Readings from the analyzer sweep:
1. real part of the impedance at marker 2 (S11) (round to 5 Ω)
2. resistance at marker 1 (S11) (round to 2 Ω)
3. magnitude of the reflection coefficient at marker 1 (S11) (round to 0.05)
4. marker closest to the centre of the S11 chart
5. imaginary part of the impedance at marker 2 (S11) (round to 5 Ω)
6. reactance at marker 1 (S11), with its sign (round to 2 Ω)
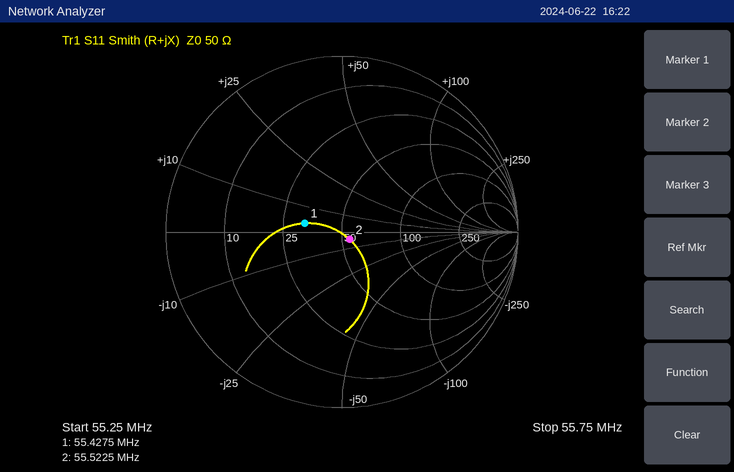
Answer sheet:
55 Ω
32 Ω
0.20
marker 2
-5 Ω
+4 Ω
